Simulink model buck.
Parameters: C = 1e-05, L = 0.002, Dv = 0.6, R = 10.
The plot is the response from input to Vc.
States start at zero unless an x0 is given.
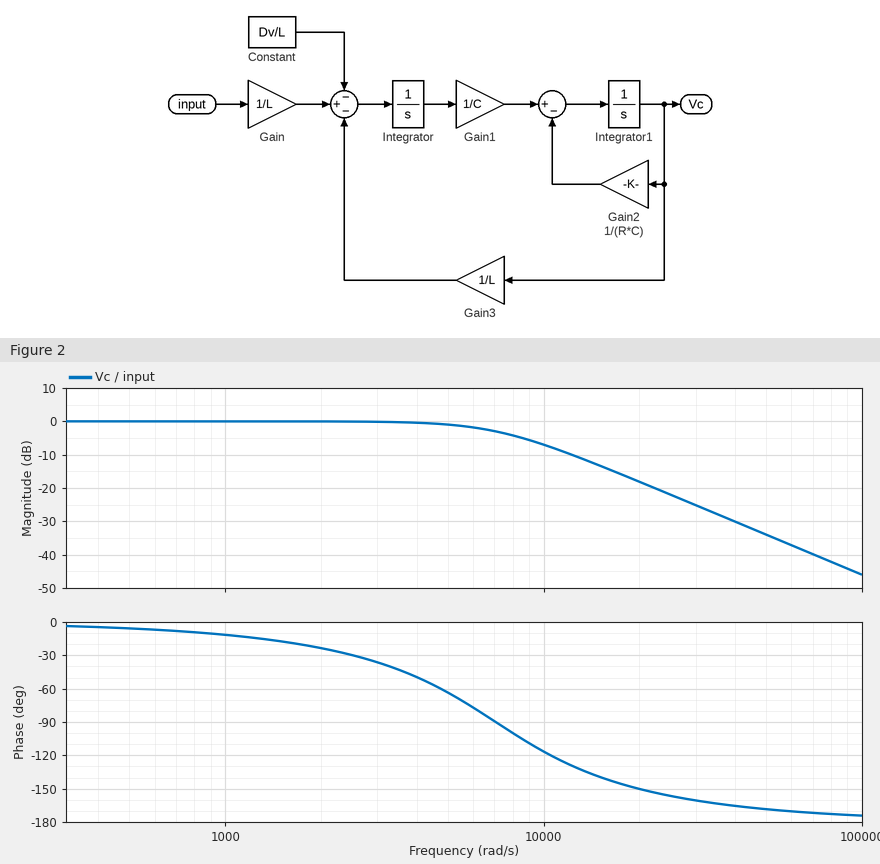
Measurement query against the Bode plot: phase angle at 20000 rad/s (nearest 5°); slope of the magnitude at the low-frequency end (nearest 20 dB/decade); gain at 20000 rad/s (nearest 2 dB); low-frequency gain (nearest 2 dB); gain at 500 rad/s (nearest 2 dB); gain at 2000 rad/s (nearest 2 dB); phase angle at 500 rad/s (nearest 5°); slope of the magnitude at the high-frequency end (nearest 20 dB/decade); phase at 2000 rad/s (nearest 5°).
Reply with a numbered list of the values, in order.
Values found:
1. -150°
2. 0 dB/decade
3. -18 dB
4. 0 dB
5. 0 dB
6. 0 dB
7. -5°
8. -40 dB/decade
9. -25°
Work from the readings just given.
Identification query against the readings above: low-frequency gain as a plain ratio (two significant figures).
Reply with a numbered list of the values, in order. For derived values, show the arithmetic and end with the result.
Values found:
1. 10^(0 / 20) = 1.0
